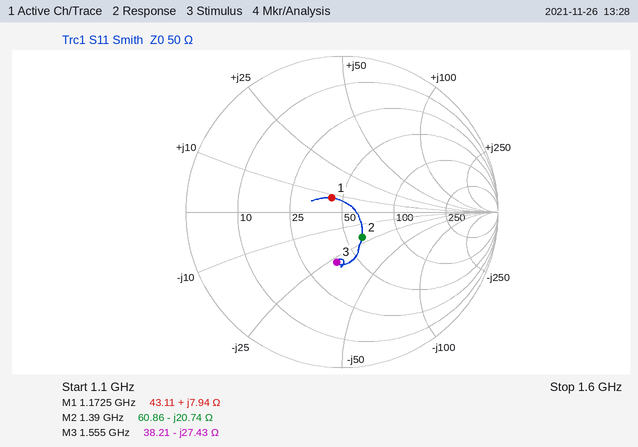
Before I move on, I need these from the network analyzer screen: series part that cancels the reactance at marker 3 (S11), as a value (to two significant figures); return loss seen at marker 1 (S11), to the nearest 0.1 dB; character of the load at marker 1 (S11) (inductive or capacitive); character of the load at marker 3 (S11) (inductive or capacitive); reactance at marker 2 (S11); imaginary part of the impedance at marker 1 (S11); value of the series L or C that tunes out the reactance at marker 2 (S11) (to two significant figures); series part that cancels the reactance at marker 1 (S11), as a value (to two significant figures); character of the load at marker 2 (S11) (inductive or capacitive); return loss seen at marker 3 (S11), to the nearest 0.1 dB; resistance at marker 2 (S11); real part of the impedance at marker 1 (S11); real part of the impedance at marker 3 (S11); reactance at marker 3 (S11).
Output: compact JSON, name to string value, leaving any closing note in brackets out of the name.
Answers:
{"series part that cancels the reactance at marker 3 (S11), as a value": "2.8 nH", "return loss seen at marker 1 (S11), to the nearest 0.1 dB": "19.0 dB", "character of the load at marker 1 (S11)": "inductive", "character of the load at marker 3 (S11)": "capacitive", "reactance at marker 2": "-20.74 Ω", "imaginary part of the impedance at marker 1": "+7.94 Ω", "value of the series L or C that tunes out the reactance at marker 2 (S11)": "2.4 nH", "series part that cancels the reactance at marker 1 (S11), as a value": "17 pF", "character of the load at marker 2 (S11)": "capacitive", "return loss seen at marker 3 (S11), to the nearest 0.1 dB": "9.8 dB", "resistance at marker 2": "60.86 Ω", "real part of the impedance at marker 1": "43.11 Ω", "real part of the impedance at marker 3": "38.21 Ω", "reactance at marker 3": "-27.43 Ω"}
